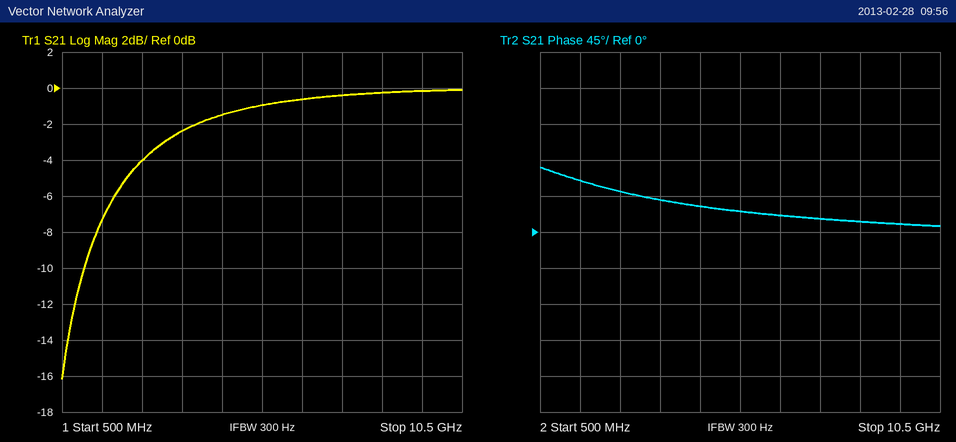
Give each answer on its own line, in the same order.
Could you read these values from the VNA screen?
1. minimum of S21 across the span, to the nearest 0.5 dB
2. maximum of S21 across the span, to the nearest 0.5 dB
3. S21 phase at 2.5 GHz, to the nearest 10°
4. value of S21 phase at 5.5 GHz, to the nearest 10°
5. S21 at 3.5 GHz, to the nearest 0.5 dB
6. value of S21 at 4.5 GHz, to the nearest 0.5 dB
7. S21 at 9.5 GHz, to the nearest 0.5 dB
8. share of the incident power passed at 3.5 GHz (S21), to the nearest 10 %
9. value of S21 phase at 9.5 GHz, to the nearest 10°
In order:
-16.0 dB
0.0 dB
50°
30°
-2.5 dB
-1.5 dB
0.0 dB
60 %
10°
